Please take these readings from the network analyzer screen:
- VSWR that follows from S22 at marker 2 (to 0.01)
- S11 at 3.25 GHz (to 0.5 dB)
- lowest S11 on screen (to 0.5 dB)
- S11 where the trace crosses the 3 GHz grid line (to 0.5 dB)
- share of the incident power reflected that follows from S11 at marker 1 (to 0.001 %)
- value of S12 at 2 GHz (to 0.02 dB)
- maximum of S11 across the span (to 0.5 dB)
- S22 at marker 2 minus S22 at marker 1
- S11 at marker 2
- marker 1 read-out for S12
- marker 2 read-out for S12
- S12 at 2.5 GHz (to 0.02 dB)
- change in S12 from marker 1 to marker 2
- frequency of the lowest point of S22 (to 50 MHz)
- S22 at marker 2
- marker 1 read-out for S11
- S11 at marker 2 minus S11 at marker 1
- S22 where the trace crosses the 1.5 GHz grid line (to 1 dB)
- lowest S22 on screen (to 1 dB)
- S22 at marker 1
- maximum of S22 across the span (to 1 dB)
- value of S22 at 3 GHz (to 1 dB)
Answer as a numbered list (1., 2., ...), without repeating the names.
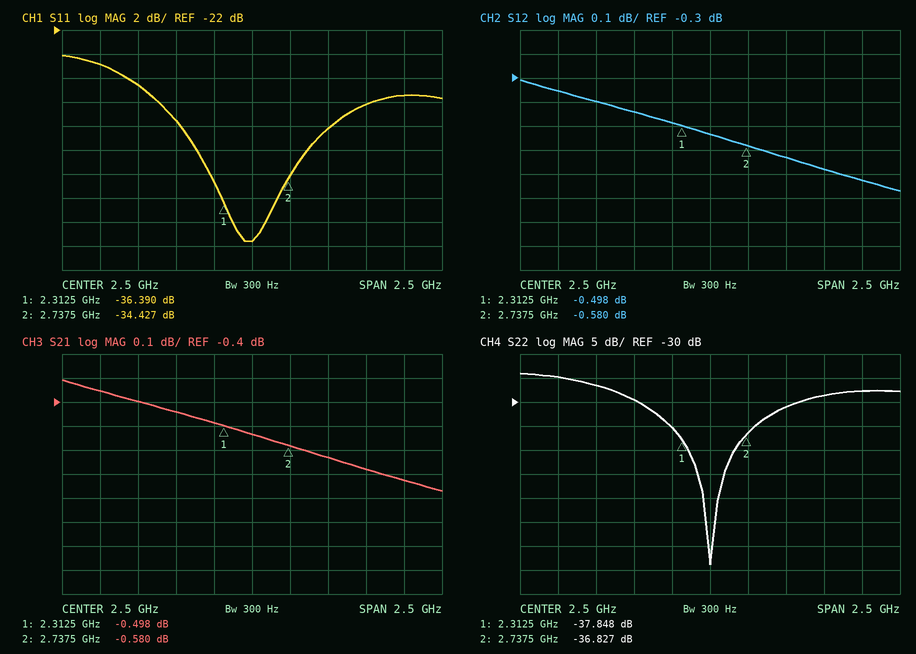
1. 1.03
2. -28.0 dB
3. -39.5 dB
4. -30.0 dB
5. 0.023 %
6. -0.44 dB
7. -24.0 dB
8. 1.021 dB
9. -34.427 dB
10. -0.498 dB
11. -0.580 dB
12. -0.54 dB
13. -0.082 dB
14. 2.50 GHz
15. -36.827 dB
16. -36.390 dB
17. 1.963 dB
18. -25 dB
19. -64 dB
20. -37.848 dB
21. -24 dB
22. -31 dB
